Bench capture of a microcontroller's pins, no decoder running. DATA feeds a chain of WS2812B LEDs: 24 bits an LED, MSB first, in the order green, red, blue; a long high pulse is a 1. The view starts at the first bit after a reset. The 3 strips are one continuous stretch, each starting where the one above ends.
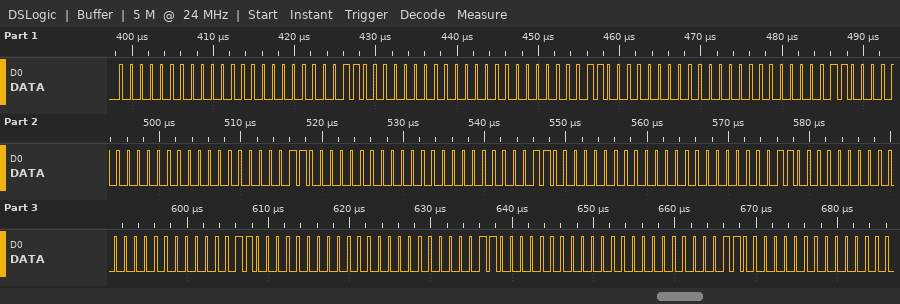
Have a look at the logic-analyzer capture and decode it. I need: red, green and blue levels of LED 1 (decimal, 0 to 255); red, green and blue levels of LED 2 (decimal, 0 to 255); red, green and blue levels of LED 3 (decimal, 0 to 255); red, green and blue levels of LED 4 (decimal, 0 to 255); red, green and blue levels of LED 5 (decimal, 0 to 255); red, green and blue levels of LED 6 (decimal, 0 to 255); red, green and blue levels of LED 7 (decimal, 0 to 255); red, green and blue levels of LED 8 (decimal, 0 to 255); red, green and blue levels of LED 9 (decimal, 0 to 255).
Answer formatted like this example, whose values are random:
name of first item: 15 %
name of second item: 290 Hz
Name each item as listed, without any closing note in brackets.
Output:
red, green and blue levels of LED 1: 0, 0, 3
red, green and blue levels of LED 2: 0, 0, 3
red, green and blue levels of LED 3: 0, 0, 3
red, green and blue levels of LED 4: 0, 0, 3
red, green and blue levels of LED 5: 0, 0, 3
red, green and blue levels of LED 6: 0, 0, 3
red, green and blue levels of LED 7: 0, 0, 3
red, green and blue levels of LED 8: 0, 0, 3
red, green and blue levels of LED 9: 0, 0, 3
